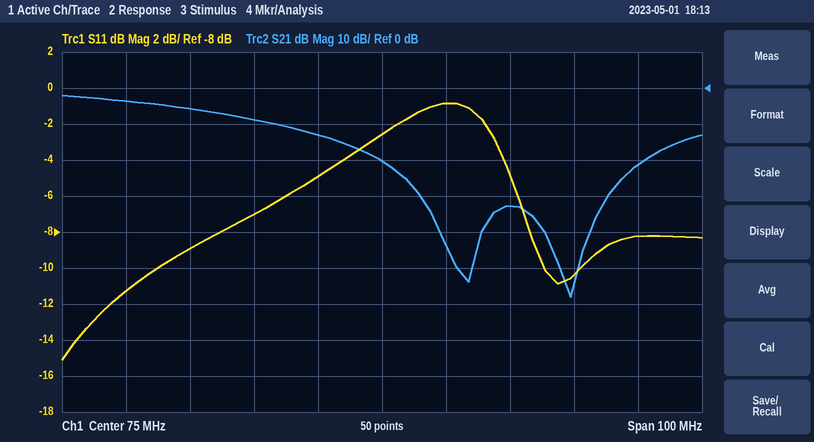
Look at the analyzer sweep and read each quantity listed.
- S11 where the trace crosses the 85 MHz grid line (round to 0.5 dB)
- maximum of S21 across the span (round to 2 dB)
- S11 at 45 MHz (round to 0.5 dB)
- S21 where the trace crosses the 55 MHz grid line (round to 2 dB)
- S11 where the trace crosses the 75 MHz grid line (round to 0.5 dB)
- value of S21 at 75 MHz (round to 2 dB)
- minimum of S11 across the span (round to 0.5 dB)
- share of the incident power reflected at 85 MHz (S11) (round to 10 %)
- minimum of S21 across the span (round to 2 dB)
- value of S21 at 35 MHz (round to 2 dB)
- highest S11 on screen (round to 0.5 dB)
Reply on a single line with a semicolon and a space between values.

-1.0 dB; -2 dB; -9.0 dB; -8 dB; -2.5 dB; -20 dB; -15.0 dB; 80 %; -58 dB; -4 dB; -1.0 dB
